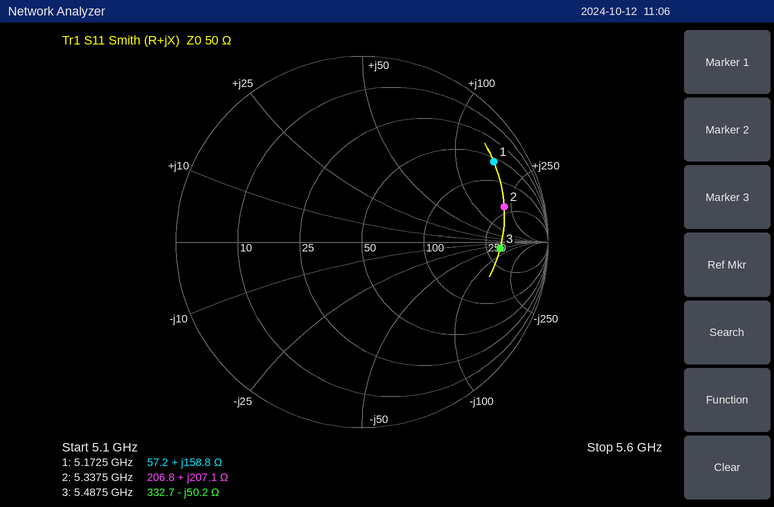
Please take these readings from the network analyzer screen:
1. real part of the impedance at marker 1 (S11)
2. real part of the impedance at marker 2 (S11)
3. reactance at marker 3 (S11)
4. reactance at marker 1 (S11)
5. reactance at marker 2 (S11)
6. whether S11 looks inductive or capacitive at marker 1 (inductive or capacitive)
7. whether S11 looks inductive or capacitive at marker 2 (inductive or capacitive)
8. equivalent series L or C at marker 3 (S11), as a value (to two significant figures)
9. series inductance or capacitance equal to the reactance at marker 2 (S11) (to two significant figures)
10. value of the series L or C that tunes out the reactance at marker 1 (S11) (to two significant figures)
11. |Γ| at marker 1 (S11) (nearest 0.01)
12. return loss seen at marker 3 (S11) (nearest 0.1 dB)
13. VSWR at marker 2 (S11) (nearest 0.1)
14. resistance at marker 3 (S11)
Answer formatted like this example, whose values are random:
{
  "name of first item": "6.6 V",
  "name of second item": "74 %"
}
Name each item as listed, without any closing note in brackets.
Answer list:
{
  "real part of the impedance at marker 1": "57.2 Ω",
  "real part of the impedance at marker 2": "206.8 Ω",
  "reactance at marker 3": "-50.2 Ω",
  "reactance at marker 1": "+158.8 Ω",
  "reactance at marker 2": "+207.1 Ω",
  "whether S11 looks inductive or capacitive at marker 1": "inductive",
  "whether S11 looks inductive or capacitive at marker 2": "inductive",
  "equivalent series L or C at marker 3 (S11), as a value": "580 fF",
  "series inductance or capacitance equal to the reactance at marker 2 (S11)": "6.2 nH",
  "value of the series L or C that tunes out the reactance at marker 1 (S11)": "190 fF",
  "|Γ| at marker 1 (S11)": "0.83",
  "return loss seen at marker 3 (S11)": "2.6 dB",
  "VSWR at marker 2 (S11)": "8.4",
  "resistance at marker 3": "332.7 Ω"
}
